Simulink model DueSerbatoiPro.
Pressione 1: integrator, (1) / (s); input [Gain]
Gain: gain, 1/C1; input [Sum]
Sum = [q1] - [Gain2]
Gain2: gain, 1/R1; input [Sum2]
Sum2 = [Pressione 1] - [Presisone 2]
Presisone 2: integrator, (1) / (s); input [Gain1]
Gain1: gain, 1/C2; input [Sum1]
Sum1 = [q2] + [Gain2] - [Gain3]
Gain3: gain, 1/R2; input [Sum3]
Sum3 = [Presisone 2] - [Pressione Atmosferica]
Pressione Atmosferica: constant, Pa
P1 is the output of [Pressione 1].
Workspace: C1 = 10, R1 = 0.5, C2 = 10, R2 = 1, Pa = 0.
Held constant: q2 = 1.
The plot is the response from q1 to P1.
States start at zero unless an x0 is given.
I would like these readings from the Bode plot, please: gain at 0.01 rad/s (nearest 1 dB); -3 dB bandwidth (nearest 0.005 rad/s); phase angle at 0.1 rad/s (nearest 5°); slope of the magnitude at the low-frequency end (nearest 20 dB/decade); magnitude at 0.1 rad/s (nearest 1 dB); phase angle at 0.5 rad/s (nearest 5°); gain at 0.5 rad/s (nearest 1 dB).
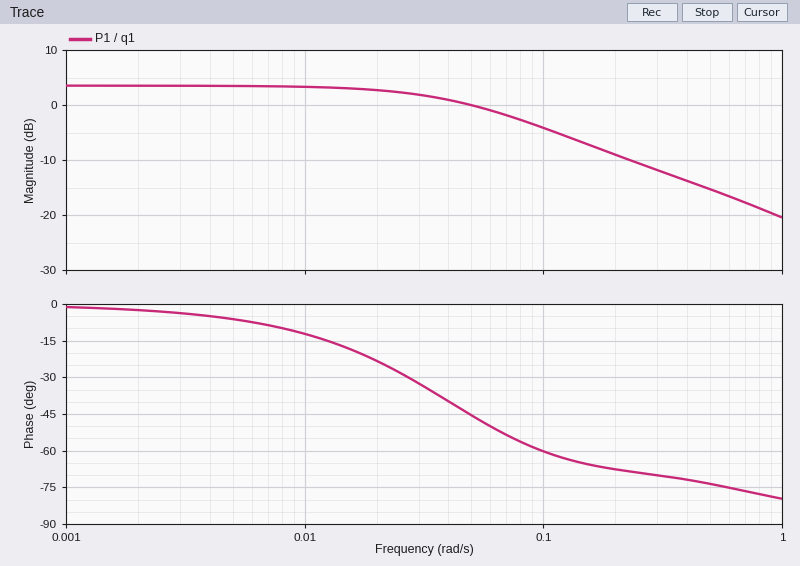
3 dB
0.045 rad/s
-60°
0 dB/decade
-4 dB
-75°
-15 dB
